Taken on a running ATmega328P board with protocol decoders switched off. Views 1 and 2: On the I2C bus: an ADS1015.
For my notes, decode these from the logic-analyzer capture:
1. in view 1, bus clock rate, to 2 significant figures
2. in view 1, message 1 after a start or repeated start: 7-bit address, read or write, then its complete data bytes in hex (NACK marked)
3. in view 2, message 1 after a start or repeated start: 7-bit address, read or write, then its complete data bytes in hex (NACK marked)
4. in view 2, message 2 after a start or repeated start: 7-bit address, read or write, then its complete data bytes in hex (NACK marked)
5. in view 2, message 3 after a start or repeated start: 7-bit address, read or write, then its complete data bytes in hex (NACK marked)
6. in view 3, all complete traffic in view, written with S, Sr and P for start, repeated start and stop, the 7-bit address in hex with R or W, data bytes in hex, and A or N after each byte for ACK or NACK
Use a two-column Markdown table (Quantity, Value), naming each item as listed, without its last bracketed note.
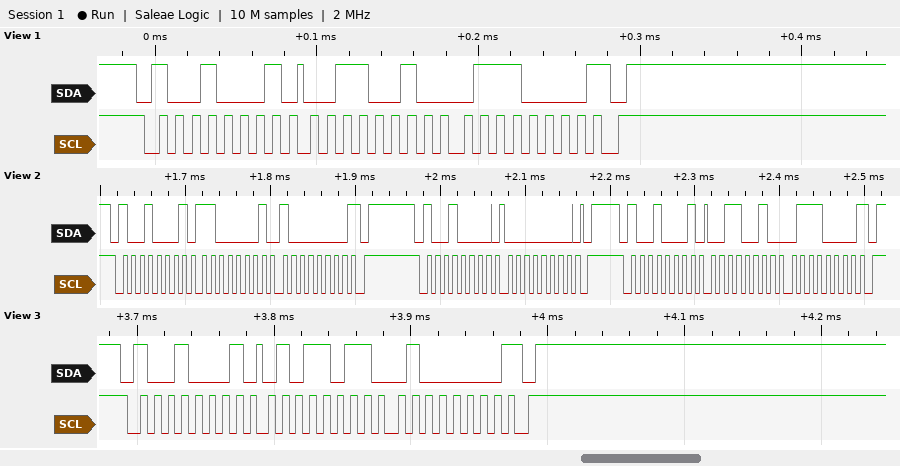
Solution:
| Quantity | Value |
|---|---|
| in view 1, bus clock rate, to 2 significant figures | 100 kHz |
| in view 1, message 1 after a start or repeated start: 7-bit address, read or write, then its complete data bytes in hex | 0x48 read: 32 70 NACK |
| in view 2, message 1 after a start or repeated start: 7-bit address, read or write, then its complete data bytes in hex | 0x48 read: C1 80 NACK |
| in view 2, message 2 after a start or repeated start: 7-bit address, read or write, then its complete data bytes in hex | 0x48 write: 00 |
| in view 2, message 3 after a start or repeated start: 7-bit address, read or write, then its complete data bytes in hex | 0x48 read: 32 70 NACK |
| in view 3, all complete traffic in view, written with S, Sr and P for start, repeated start and stop, the 7-bit address in hex with R or W, data bytes in hex, and A or N after each byte for ACK or NACK | S 48R A 5B A 40 N P |
